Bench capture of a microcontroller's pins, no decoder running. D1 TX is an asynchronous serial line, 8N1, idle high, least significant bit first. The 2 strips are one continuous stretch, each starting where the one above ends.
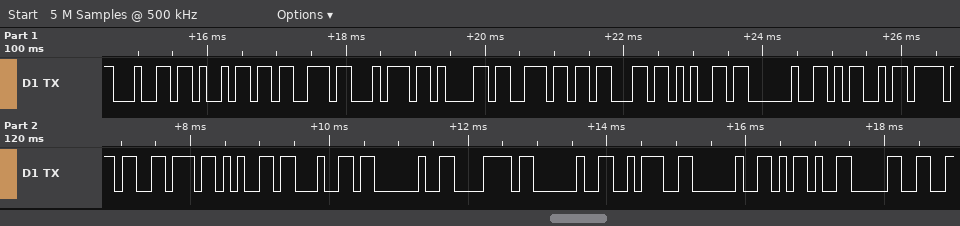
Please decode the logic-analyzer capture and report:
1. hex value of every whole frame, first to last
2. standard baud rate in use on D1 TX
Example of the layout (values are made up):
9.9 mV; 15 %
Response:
64 69 73 74 61 6E 63 65 20 4D 6F 76 65 64 20 78 20 3A 20 2D 30; 9600 baud
